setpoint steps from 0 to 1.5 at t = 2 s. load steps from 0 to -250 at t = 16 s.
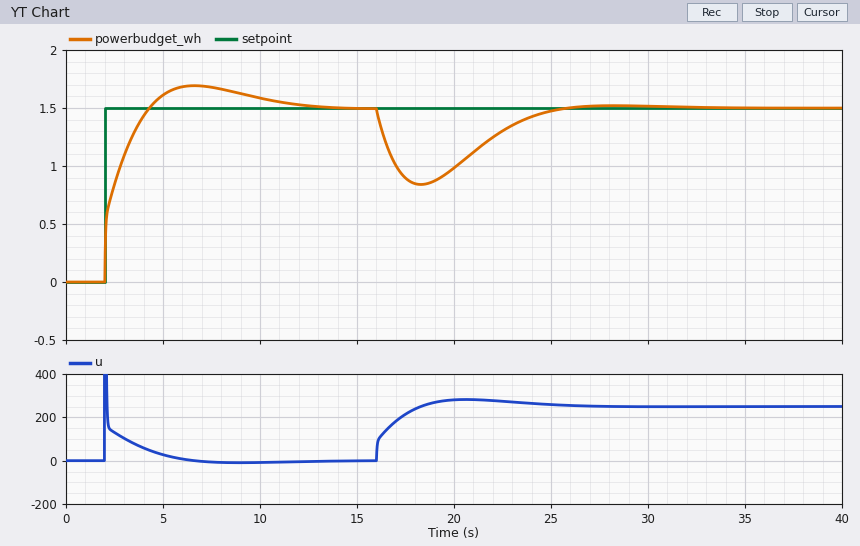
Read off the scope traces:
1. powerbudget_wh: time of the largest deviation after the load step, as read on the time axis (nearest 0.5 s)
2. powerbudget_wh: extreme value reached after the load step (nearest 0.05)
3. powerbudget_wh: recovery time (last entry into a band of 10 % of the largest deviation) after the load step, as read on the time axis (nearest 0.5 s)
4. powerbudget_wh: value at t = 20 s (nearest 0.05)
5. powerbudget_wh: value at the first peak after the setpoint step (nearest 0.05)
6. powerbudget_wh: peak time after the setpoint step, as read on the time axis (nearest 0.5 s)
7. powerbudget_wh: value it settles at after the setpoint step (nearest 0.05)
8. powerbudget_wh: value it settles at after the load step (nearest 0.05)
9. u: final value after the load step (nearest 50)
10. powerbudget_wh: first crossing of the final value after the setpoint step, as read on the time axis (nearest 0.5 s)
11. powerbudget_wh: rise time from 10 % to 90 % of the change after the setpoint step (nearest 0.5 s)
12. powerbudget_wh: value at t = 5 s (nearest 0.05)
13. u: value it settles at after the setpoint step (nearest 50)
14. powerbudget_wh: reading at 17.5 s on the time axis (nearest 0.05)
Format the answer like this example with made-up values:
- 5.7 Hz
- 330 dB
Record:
- 18.5 s
- 0.85
- 24.0 s
- 1.00
- 1.70
- 6.5 s
- 1.50
- 1.50
- 250
- 4.5 s
- 1.5 s
- 1.60
- 0
- 0.90
